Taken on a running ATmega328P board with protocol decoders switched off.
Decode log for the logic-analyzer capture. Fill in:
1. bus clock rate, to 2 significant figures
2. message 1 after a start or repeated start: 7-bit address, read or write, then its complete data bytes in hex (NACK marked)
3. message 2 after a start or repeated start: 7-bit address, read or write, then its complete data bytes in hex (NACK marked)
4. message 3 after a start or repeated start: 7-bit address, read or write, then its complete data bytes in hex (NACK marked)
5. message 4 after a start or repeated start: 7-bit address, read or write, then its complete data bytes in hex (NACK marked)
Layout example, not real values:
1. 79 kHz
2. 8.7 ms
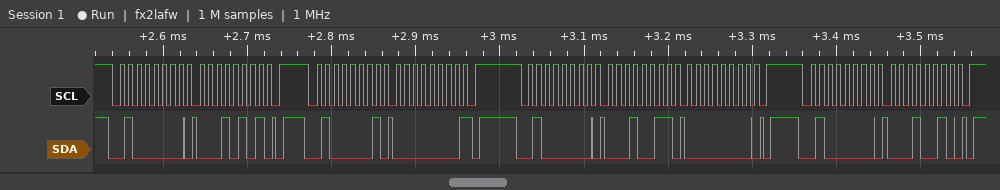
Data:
1. 100 kHz
2. 0x20 write: 15
3. 0x20 read: 00 NACK
4. 0x20 write: 13 00
5. 0x20 write: 12
